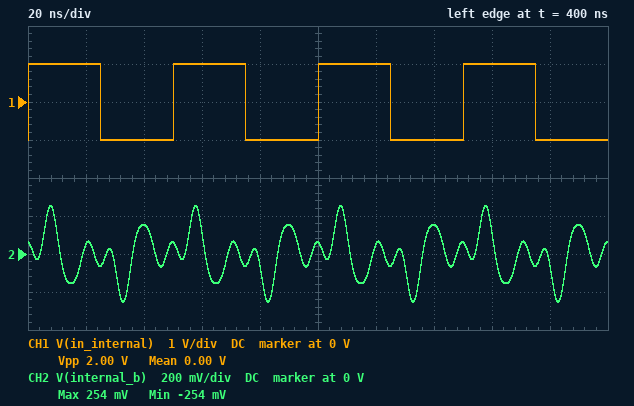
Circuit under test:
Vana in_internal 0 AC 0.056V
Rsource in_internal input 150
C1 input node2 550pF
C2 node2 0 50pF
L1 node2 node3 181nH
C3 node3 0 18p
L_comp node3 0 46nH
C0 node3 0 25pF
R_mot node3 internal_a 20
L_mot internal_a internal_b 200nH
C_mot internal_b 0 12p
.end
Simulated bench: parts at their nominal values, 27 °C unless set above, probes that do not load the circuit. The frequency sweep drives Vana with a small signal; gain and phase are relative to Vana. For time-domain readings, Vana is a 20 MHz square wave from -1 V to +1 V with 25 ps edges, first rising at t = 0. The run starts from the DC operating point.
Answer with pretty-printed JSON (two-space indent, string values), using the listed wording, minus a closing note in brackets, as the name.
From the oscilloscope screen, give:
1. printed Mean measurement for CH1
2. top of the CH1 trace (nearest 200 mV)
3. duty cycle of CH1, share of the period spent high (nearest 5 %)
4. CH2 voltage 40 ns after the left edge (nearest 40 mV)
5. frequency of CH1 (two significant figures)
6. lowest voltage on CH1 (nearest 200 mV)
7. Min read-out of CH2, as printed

{
  "printed Mean measurement for CH1": "0.00 V",
  "top of the CH1 trace": "1.0 V",
  "duty cycle of CH1, share of the period spent high": "50 %",
  "CH2 voltage 40 ns after the left edge": "160 mV",
  "frequency of CH1": "20 MHz",
  "lowest voltage on CH1": "-1.0 V",
  "Min read-out of CH2, as printed": "-254 mV"
}
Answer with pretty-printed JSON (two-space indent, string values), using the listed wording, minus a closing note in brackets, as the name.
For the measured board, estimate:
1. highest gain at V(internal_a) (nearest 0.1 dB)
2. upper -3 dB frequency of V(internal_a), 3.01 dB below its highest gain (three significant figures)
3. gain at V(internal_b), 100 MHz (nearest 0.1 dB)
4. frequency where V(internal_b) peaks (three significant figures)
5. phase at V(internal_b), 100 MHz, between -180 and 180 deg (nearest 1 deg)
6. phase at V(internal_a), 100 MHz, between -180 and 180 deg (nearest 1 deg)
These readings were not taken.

{
  "highest gain at V(internal_a)": "-7.3 dB",
  "upper -3 dB frequency of V(internal_a), 3.01 dB below its highest gain": "152 MHz",
  "gain at V(internal_b), 100 MHz": "-9.4 dB",
  "frequency where V(internal_b) peaks": "89.6 MHz",
  "phase at V(internal_b), 100 MHz, between -180 and 180 deg": "132 deg",
  "phase at V(internal_a), 100 MHz, between -180 and 180 deg": "132 deg"
}
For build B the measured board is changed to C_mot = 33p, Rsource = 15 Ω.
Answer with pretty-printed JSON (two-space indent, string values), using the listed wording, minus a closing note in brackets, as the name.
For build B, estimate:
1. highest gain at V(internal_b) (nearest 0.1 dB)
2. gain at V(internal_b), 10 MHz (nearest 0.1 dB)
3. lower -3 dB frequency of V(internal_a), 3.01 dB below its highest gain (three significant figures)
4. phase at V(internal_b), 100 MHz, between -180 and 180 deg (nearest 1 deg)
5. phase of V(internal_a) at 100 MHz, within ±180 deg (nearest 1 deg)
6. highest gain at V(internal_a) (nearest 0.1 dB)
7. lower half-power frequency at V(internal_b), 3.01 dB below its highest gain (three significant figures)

{
  "highest gain at V(internal_b)": "0.1 dB",
  "gain at V(internal_b), 10 MHz": "-16.3 dB",
  "lower -3 dB frequency of V(internal_a), 3.01 dB below its highest gain": "138 MHz",
  "phase at V(internal_b), 100 MHz, between -180 and 180 deg": "169 deg",
  "phase of V(internal_a) at 100 MHz, within ±180 deg": "-11 deg",
  "highest gain at V(internal_a)": "11.4 dB",
  "lower half-power frequency at V(internal_b), 3.01 dB below its highest gain": "48.6 MHz"
}
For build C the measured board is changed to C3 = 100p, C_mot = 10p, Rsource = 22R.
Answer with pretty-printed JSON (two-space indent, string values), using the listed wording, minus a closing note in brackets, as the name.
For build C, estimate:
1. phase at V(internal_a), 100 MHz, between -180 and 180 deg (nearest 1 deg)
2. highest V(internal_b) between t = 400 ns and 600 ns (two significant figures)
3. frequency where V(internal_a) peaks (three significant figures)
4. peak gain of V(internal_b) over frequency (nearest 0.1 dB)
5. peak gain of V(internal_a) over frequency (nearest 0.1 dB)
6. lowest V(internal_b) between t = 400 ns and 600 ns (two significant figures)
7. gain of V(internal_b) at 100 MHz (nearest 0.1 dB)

{
  "phase at V(internal_a), 100 MHz, between -180 and 180 deg": "138 deg",
  "highest V(internal_b) between t = 400 ns and 600 ns": "710 mV",
  "frequency where V(internal_a) peaks": "70.6 MHz",
  "peak gain of V(internal_b) over frequency": "13.4 dB",
  "peak gain of V(internal_a) over frequency": "9.1 dB",
  "lowest V(internal_b) between t = 400 ns and 600 ns": "-710 mV",
  "gain of V(internal_b) at 100 MHz": "-5.6 dB"
}
